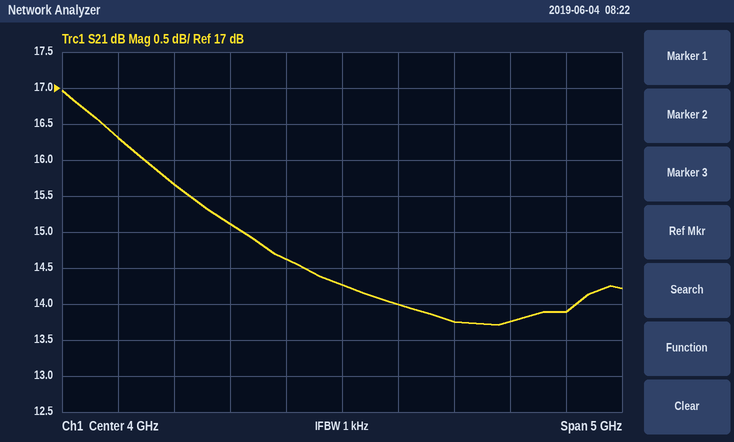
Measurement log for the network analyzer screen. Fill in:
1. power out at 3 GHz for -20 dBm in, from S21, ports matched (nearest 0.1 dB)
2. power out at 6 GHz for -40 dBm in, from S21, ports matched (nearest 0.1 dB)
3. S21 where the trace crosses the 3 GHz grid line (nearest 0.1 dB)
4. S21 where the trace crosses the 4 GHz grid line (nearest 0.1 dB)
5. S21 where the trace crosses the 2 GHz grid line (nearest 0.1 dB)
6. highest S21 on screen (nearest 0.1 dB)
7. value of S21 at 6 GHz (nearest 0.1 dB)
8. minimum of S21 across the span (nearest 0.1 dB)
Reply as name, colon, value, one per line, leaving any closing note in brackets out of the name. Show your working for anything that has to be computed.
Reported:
power out at 3 GHz for -20 dBm in, from S21, ports matched: -20 dBm + (15.1 dB) = -4.9 dBm
power out at 6 GHz for -40 dBm in, from S21, ports matched: -40 dBm + (13.9 dB) = -26.1 dBm
S21 where the trace crosses the 3 GHz grid line: 15.1 dB
S21 where the trace crosses the 4 GHz grid line: 14.3 dB
S21 where the trace crosses the 2 GHz grid line: 16.3 dB
highest S21 on screen: 17.0 dB
value of S21 at 6 GHz: 13.9 dB
minimum of S21 across the span: 13.7 dB
